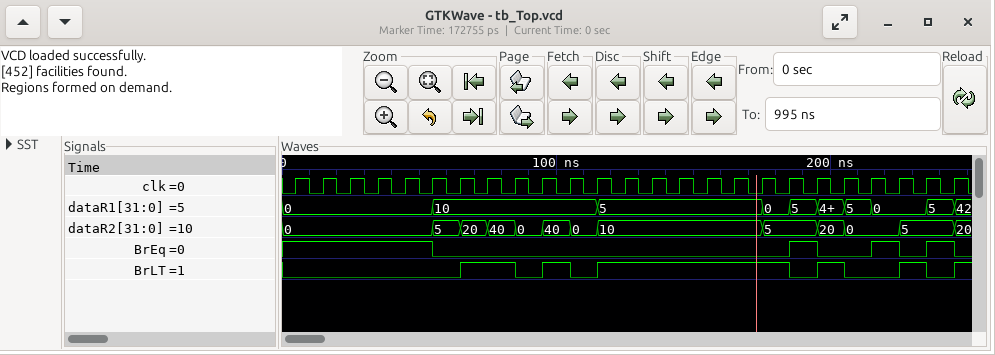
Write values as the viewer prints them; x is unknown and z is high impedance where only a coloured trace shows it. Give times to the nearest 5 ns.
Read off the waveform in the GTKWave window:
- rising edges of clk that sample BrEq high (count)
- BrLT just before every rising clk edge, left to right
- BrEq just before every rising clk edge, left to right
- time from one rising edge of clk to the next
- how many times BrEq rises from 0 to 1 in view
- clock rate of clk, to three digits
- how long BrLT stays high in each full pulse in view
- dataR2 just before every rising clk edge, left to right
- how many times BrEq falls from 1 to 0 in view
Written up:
9
0 0 0 0 0 0 0 1 1 0 1 0 1 1 1 1 1 1 1 0 1 0 0 1 0
1 1 1 1 1 1 0 0 0 0 0 0 0 0 0 0 0 0 0 1 0 0 1 0 1
10 ns
3
100 MHz
20 ns, 10 ns, 70 ns, 10 ns, 10 ns
0, 0, 0, 0, 0, 0, 5, 20, 40, 0, 40, 0, 10, 10, 10, 10, 10, 10, 5, 5, 20, 0, 0, 5, 5
4
